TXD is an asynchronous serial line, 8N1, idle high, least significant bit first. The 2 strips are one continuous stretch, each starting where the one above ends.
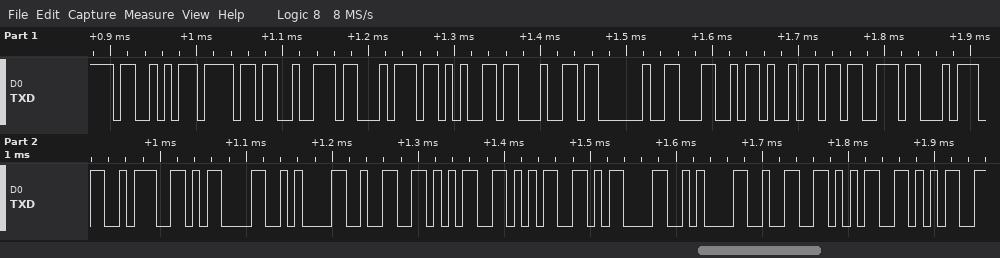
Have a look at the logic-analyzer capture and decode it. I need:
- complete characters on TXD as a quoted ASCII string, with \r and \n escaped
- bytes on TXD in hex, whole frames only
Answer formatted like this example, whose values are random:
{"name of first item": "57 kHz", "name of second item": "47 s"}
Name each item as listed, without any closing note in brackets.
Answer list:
{"complete characters on TXD as a quoted ASCII string, with \\r and \\n escaped": "\"Sorted List:\\r\\n255\\r\\n255\"", "bytes on TXD in hex, whole frames only": "53 6F 72 74 65 64 20 4C 69 73 74 3A 0D 0A 32 35 35 0D 0A 32 35 35"}
